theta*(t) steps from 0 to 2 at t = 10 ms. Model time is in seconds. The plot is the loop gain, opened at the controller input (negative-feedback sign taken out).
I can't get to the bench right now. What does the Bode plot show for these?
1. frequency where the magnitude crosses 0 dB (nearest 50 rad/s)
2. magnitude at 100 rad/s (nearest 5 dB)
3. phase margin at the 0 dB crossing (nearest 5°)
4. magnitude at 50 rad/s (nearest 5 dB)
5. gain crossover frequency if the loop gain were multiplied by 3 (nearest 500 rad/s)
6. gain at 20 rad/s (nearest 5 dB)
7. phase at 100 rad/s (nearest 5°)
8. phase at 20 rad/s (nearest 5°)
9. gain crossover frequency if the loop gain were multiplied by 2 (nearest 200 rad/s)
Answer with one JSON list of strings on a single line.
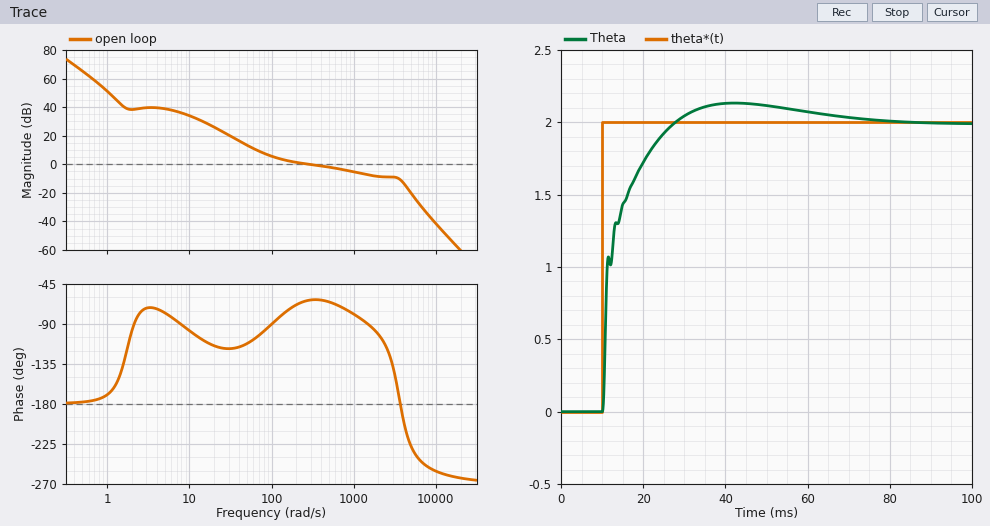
["300 rad/s", "5 dB", "115°", "15 dB", "3500 rad/s", "25 dB", "-90°", "-115°", "1200 rad/s"]
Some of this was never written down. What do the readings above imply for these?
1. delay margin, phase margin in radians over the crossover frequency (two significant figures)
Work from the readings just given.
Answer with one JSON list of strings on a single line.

["0.0067 s"]
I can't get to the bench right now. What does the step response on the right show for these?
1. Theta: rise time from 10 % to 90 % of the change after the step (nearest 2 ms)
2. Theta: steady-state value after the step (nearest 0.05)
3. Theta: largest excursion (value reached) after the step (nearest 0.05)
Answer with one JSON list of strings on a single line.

["12 ms", "2.00", "2.15"]
